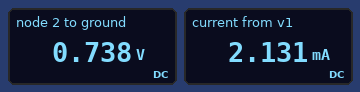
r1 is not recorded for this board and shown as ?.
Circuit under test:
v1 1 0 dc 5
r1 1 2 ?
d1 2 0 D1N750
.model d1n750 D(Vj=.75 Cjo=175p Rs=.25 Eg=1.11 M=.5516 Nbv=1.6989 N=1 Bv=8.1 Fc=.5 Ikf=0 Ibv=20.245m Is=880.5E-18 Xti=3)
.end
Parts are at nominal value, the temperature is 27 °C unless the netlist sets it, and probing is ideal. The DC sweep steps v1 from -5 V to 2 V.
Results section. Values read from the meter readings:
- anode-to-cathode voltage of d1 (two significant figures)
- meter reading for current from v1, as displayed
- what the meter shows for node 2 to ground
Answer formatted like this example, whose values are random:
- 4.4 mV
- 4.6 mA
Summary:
- 740 mV
- 2.131 mA
- 0.738 V
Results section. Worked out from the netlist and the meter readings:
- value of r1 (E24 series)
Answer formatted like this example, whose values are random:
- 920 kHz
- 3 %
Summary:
- 2 kΩ
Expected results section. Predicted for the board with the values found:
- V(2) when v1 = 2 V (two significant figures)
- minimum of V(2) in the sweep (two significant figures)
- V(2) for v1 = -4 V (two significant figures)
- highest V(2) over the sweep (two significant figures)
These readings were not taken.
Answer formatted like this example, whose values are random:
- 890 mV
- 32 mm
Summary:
- 710 mV
- -5.0 V
- -4.0 V
- 710 mV
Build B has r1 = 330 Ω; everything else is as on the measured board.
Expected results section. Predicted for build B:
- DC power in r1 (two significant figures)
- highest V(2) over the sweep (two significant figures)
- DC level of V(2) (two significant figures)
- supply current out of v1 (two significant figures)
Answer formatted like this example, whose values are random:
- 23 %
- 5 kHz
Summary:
- 54 mW
- 750 mV
- 790 mV
- 13 mA
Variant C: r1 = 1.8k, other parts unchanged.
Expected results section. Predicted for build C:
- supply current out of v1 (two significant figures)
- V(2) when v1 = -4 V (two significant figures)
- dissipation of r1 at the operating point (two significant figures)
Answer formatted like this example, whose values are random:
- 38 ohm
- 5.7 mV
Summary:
- 2.4 mA
- -4.0 V
- 10 mW
